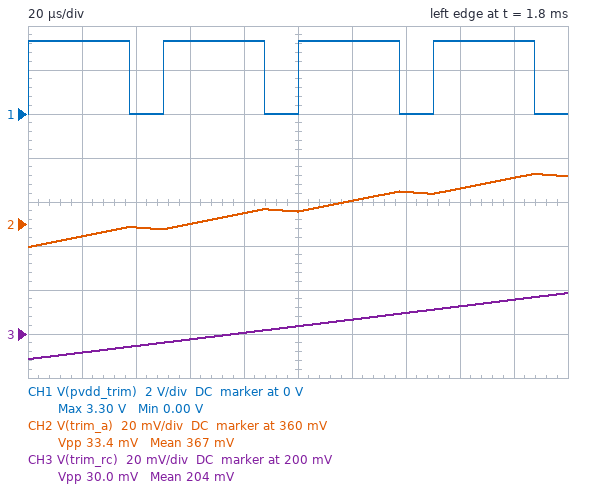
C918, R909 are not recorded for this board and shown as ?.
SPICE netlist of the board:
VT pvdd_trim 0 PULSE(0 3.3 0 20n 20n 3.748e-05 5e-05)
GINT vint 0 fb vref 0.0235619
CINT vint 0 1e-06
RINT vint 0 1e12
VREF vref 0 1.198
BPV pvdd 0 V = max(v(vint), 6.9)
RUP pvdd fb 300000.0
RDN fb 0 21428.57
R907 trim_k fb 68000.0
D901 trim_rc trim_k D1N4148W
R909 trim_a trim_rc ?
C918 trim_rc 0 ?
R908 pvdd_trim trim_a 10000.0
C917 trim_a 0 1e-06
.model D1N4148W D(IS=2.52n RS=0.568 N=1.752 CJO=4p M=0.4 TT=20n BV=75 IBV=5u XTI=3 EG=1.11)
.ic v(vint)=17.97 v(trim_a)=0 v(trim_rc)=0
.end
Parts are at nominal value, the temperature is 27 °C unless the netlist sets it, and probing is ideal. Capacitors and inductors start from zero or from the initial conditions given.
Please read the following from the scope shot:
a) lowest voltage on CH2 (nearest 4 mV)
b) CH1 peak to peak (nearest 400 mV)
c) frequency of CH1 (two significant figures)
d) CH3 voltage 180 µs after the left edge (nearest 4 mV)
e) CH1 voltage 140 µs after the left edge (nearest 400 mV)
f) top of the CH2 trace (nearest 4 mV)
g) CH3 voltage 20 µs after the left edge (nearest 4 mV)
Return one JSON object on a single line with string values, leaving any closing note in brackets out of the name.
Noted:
{"lowest voltage on CH2": "348 mV", "CH1 peak to peak": "3.2 V", "frequency of CH1": "20 kHz", "CH3 voltage 180 µs after the left edge": "216 mV", "CH1 voltage 140 µs after the left edge": "0 V", "top of the CH2 trace": "384 mV", "CH3 voltage 20 µs after the left edge": "192 mV"}
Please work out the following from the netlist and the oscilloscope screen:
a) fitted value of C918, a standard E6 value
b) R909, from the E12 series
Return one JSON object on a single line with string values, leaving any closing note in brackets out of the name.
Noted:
{"fitted value of C918, a standard E6 value": "330 nF", "R909, from the E12 series": "3.3 kΩ"}
